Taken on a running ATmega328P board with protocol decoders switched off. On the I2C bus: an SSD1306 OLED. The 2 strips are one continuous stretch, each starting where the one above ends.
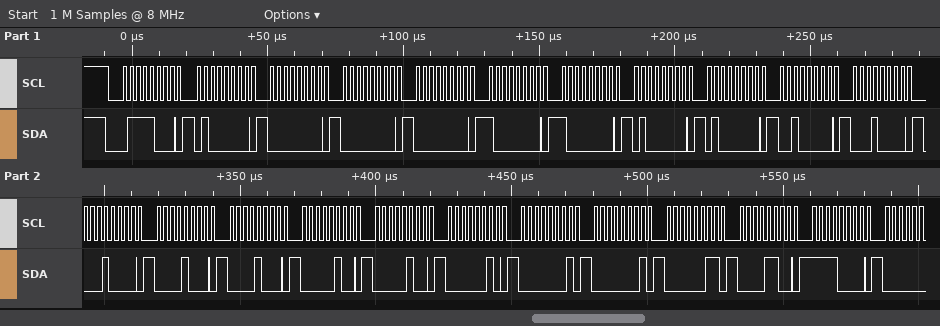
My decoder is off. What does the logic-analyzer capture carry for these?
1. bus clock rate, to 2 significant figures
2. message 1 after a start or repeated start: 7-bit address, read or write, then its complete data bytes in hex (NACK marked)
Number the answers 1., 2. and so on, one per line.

1. 400 kHz
2. 0x3C write: 40 00 00 00 80 80 40 40 20 10 10 08 08 04 04 02 01 01 03 0C F0
